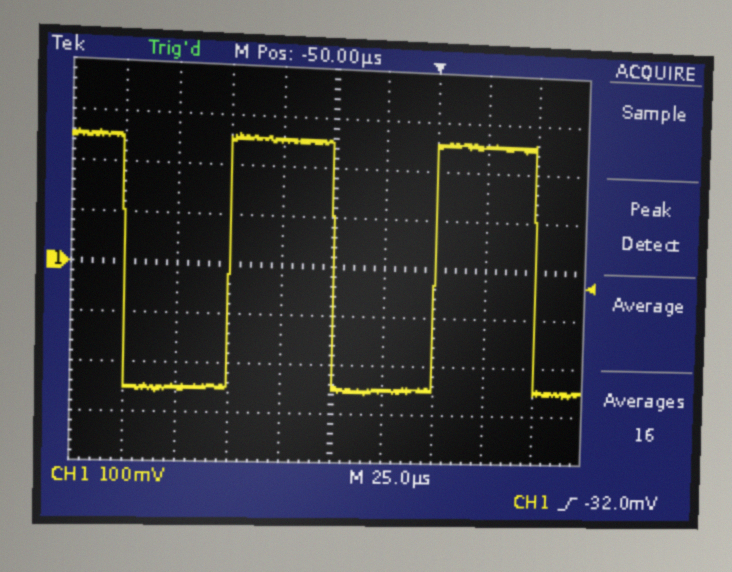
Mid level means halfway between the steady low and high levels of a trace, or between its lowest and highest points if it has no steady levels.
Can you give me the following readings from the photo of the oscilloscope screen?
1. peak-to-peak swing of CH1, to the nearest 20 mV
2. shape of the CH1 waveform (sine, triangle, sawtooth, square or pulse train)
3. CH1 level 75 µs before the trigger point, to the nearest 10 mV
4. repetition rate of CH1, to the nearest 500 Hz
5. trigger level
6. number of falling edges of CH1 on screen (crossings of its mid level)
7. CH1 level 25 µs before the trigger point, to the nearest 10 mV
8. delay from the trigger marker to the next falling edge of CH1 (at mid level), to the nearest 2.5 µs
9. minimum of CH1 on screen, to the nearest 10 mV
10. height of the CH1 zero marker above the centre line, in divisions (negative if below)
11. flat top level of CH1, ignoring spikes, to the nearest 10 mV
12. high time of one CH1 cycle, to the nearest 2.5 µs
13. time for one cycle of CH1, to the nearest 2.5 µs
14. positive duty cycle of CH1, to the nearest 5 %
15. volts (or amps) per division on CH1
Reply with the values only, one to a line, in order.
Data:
520 mV
square
250 mV
10.0 kHz
-32.0 mV
3
-250 mV
50.0 µs
-260 mV
0.0 div
250 mV
50.0 µs
100.0 µs
50 %
100 mV
